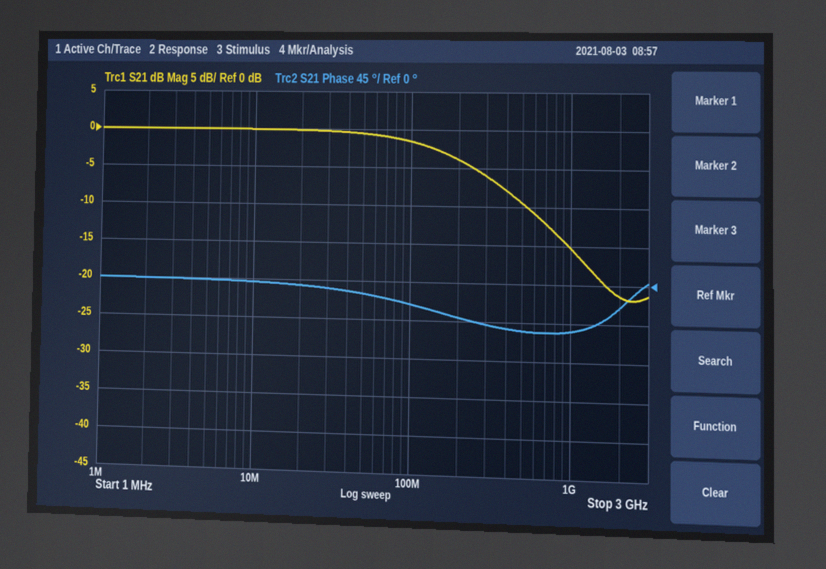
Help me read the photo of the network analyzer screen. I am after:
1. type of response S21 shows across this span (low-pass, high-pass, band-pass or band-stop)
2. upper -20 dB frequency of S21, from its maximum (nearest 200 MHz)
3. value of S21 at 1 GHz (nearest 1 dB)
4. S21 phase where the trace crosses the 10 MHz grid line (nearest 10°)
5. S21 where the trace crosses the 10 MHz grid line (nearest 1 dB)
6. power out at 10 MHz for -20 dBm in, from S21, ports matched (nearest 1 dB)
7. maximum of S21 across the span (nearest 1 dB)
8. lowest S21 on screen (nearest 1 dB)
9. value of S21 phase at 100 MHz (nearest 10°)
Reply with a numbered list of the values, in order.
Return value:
1. low-pass
2. 1.6 GHz
3. -15 dB
4. 0°
5. 0 dB
6. -20 dBm
7. 0 dB
8. -22 dB
9. -30°
